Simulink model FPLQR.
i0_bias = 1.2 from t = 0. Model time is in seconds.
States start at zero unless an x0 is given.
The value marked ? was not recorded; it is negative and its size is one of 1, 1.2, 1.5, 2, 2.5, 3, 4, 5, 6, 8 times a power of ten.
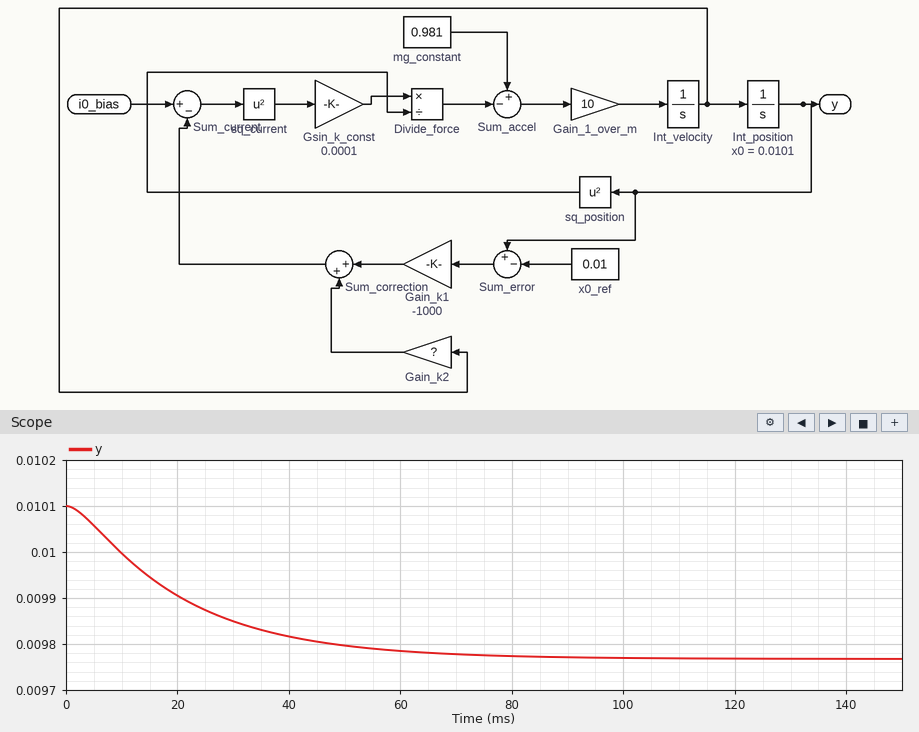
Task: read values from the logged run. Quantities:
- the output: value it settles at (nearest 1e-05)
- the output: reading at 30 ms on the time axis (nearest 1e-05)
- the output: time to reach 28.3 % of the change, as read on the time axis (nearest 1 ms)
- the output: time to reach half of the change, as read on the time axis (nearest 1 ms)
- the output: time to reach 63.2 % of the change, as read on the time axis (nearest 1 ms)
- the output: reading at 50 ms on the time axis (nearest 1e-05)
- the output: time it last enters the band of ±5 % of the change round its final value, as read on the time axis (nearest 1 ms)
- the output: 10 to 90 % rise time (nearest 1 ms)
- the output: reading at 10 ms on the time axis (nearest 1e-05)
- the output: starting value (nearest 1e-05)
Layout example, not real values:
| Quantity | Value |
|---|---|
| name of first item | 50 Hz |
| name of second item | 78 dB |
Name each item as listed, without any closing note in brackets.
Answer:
| Quantity | Value |
|---|---|
| the output: value it settles at | 0.00977 |
| the output: reading at 30 ms on the time axis | 0.00985 |
| the output: time to reach 28.3 % of the change, as read on the time axis | 9 ms |
| the output: time to reach half of the change, as read on the time axis | 16 ms |
| the output: time to reach 63.2 % of the change, as read on the time axis | 22 ms |
| the output: reading at 50 ms on the time axis | 0.00980 |
| the output: time it last enters the band of ±5 % of the change round its final value, as read on the time axis | 61 ms |
| the output: 10 to 90 % rise time | 43 ms |
| the output: reading at 10 ms on the time axis | 0.01000 |
| the output: starting value | 0.01010 |
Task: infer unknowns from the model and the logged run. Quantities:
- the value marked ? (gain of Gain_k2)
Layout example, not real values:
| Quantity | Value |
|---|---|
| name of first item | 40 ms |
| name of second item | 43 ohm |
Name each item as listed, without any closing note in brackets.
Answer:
| Quantity | Value |
|---|---|
| the value marked ? | -20 |
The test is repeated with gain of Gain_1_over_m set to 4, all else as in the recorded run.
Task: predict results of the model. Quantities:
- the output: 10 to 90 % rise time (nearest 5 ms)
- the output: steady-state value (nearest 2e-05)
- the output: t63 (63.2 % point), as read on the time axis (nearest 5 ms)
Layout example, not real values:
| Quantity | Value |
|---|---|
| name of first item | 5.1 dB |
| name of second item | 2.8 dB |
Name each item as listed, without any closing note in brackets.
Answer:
| Quantity | Value |
|---|---|
| the output: 10 to 90 % rise time | 35 ms |
| the output: steady-state value | 0.00976 |
| the output: t63 (63.2 % point), as read on the time axis | 25 ms |
